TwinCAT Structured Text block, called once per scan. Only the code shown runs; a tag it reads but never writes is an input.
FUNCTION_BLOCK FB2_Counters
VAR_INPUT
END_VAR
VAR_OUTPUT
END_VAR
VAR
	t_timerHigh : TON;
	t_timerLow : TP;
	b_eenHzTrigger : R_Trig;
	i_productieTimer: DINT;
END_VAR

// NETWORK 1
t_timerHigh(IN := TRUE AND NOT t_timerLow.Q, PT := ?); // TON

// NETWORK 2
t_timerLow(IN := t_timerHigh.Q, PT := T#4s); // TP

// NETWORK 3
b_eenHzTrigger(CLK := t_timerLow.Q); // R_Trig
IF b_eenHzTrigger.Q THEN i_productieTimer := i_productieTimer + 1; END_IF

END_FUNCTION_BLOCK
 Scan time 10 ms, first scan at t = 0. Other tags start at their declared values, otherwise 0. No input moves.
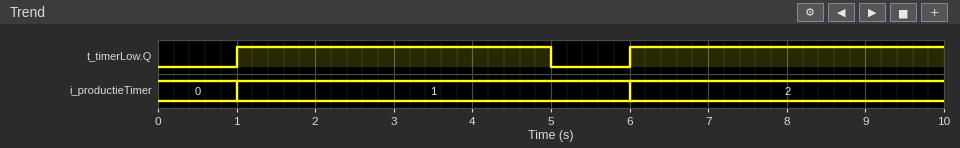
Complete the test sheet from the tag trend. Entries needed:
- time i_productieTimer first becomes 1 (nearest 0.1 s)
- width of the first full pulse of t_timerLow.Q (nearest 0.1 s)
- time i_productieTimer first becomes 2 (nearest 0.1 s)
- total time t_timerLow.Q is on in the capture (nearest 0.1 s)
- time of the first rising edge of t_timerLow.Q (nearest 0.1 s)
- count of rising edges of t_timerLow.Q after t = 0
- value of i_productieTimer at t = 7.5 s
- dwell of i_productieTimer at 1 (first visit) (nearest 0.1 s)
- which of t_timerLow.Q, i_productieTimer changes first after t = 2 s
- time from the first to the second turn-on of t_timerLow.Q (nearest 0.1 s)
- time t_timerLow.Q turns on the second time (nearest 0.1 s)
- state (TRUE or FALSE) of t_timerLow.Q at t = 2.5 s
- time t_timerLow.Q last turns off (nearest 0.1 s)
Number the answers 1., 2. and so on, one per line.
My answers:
1. 1.0 s
2. 4.0 s
3. 6.0 s
4. 8.0 s
5. 1.0 s
6. 2
7. 2
8. 5.0 s
9. t_timerLow.Q
10. 5.0 s
11. 6.0 s
12. TRUE
13. 5.0 s
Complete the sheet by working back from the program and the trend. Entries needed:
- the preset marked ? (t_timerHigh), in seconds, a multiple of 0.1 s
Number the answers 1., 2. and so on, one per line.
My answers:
1. 1.0 s
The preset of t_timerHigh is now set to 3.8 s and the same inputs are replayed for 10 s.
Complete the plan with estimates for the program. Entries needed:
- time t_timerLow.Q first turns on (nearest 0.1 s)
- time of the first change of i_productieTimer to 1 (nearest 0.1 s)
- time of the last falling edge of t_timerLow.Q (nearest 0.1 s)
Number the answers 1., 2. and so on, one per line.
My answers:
1. 3.8 s
2. 3.8 s
3. 7.8 s
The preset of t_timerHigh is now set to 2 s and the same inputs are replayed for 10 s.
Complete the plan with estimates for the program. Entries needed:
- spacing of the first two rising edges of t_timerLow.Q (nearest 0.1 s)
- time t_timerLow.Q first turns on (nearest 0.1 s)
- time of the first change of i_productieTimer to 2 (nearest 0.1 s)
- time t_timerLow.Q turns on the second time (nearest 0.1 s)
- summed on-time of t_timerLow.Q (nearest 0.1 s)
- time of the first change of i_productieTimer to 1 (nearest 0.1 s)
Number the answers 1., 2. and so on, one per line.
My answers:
1. 6.0 s
2. 2.0 s
3. 8.0 s
4. 8.0 s
5. 6.0 s
6. 2.0 s
